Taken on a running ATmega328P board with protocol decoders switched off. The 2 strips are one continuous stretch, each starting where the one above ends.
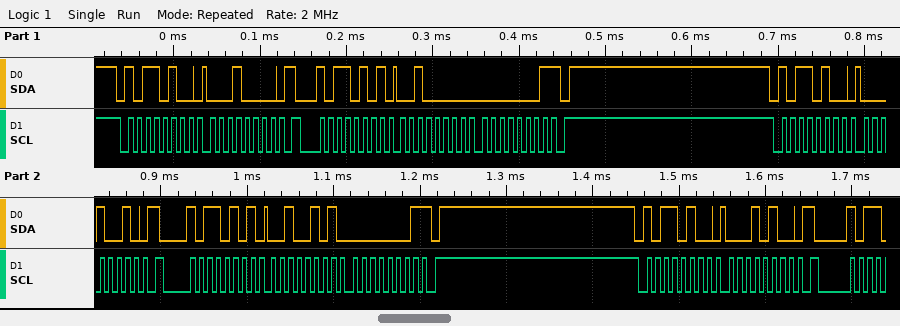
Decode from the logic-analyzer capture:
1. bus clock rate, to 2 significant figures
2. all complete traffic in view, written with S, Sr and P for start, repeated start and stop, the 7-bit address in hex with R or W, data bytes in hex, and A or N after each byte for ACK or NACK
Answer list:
100 kHz
S 5AW A 10 A Sr 5AR A 20 A 01 N P S 5AW A 12 A Sr 5AR A 25 A 01 N P S 5AW A 14 A
